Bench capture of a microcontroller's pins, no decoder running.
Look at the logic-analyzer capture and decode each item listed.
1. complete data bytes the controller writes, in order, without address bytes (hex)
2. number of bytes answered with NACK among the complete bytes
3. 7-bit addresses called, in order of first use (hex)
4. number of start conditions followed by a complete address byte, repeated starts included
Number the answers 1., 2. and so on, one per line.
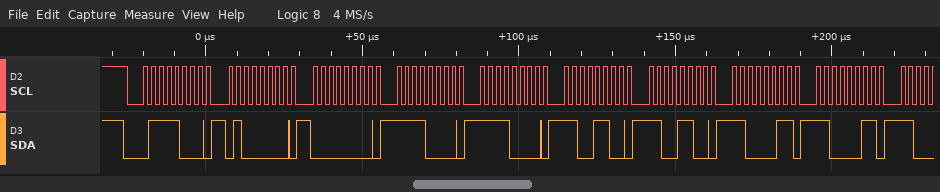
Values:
1. 40 00 F0 F0 CC CC C3 C3
2. 0
3. 0x3C
4. 1
